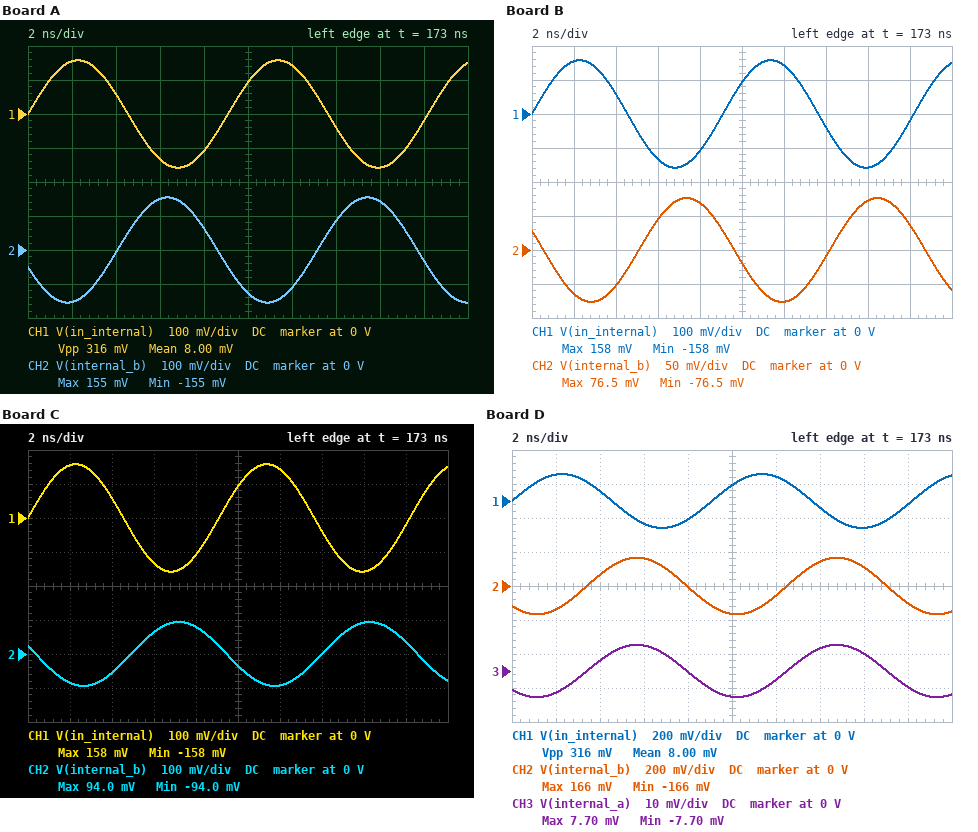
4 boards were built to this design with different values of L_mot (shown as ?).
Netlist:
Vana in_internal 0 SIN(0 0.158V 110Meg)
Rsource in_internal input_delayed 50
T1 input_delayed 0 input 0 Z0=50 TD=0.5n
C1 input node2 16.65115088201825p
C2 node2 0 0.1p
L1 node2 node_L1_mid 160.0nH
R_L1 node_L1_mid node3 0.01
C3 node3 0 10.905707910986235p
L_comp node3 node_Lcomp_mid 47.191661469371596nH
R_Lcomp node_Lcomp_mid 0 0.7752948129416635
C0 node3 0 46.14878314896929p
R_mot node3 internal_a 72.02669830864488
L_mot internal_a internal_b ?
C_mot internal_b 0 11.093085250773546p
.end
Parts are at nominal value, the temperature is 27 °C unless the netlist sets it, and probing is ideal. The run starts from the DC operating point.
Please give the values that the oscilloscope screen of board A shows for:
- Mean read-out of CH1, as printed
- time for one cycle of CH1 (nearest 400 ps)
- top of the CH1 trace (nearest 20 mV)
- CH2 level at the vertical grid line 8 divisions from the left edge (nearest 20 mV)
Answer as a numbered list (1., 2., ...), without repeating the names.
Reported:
1. 8.00 mV
2. 9.2 ns
3. 160 mV
4. 140 mV
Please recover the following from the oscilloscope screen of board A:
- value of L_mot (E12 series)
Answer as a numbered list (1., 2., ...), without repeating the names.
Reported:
1. 270 nH
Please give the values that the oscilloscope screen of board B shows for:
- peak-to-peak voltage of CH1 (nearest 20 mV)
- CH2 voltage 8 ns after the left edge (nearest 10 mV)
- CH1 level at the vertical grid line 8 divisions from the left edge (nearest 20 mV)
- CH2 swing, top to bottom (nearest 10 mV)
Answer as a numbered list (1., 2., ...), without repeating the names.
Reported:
1. 320 mV
2. 70 mV
3. -160 mV
4. 150 mV
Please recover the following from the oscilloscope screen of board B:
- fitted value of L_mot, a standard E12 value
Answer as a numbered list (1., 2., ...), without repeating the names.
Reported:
1. 560 nH
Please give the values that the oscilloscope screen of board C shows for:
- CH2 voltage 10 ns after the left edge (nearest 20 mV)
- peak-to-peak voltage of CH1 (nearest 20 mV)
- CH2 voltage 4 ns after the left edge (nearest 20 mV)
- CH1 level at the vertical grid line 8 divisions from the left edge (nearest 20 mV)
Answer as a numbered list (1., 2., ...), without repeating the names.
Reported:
1. -40 mV
2. 320 mV
3. -60 mV
4. -160 mV
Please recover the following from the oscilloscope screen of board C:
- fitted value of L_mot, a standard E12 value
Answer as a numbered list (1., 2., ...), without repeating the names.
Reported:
1. 470 nH
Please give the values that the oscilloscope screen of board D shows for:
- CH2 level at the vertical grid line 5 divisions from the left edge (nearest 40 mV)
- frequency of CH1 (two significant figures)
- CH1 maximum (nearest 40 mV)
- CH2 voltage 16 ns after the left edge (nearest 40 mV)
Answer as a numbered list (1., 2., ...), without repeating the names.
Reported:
1. -160 mV
2. 110 MHz
3. 160 mV
4. 120 mV
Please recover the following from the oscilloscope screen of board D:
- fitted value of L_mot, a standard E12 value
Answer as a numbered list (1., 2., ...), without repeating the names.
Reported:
1. 180 nH
